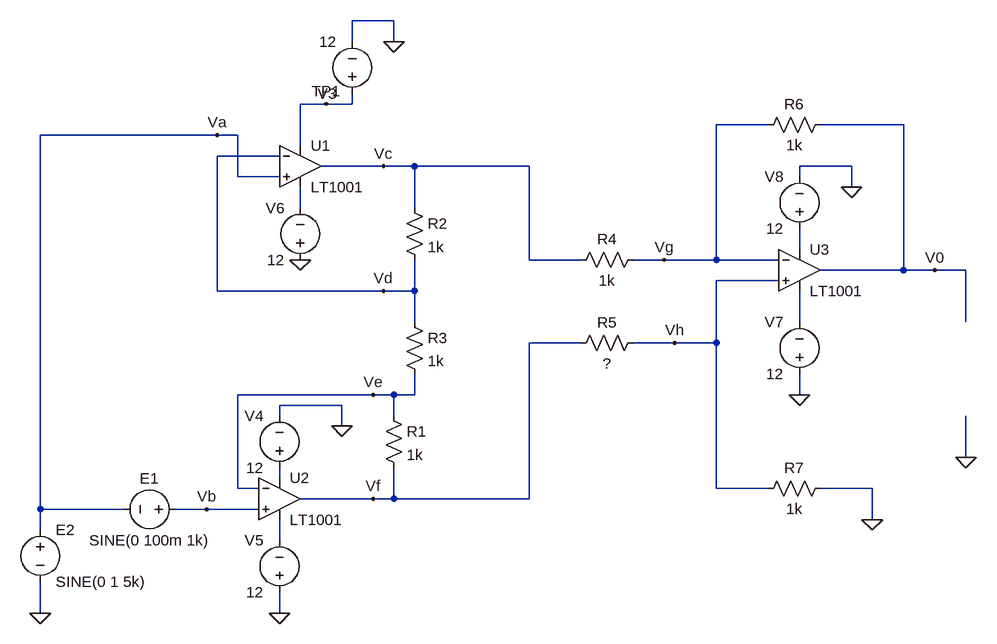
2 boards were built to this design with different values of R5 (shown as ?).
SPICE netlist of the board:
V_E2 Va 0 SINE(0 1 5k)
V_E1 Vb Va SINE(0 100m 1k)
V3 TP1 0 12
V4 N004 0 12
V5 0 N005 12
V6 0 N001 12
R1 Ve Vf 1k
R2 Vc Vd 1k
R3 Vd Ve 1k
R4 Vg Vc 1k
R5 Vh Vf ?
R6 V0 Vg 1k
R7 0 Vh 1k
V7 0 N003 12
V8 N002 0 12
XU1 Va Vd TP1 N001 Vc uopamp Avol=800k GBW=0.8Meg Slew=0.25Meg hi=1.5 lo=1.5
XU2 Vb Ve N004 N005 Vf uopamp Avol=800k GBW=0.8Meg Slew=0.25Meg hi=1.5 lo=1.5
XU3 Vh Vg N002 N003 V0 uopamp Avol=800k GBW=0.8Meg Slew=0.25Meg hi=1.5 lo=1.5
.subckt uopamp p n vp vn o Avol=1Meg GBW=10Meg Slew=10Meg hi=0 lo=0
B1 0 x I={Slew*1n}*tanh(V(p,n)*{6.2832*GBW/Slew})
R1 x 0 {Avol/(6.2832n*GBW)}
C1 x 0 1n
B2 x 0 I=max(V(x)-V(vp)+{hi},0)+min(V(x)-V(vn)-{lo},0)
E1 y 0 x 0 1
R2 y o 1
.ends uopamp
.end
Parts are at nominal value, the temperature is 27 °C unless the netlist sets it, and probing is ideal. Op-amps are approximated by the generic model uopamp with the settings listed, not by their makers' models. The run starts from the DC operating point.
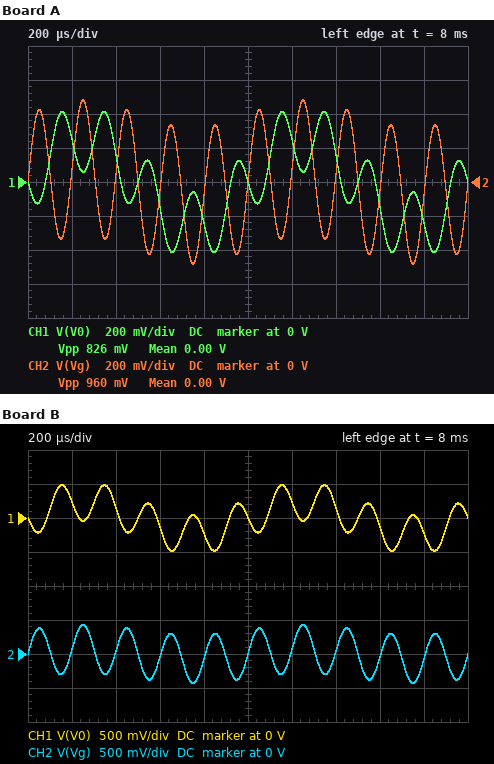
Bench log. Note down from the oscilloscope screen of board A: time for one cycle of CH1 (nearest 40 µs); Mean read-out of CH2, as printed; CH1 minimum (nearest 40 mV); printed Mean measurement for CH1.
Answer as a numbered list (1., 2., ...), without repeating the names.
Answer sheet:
1. 1.00 ms
2. 0.00 V
3. -400 mV
4. 0.00 V
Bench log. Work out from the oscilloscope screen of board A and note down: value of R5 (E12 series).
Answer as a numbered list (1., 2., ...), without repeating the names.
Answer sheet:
1. 1.5 kΩ
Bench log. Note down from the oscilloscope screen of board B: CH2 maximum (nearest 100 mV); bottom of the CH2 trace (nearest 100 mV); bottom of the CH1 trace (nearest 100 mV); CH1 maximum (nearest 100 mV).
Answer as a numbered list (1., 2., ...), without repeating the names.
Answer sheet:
1. 400 mV
2. -400 mV
3. -500 mV
4. 500 mV
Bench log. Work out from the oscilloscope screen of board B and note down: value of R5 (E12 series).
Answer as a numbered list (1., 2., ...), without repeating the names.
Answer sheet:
1. 1.8 kΩ
